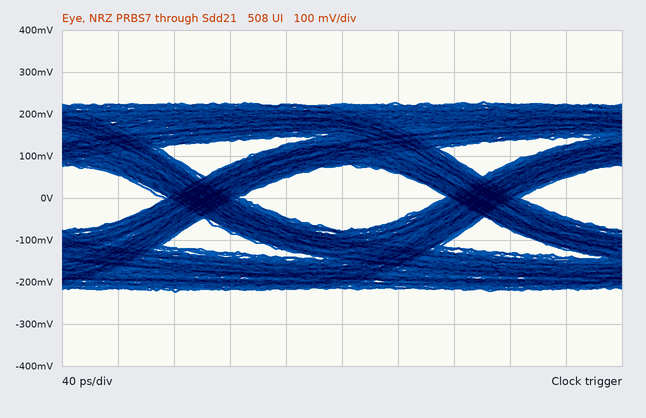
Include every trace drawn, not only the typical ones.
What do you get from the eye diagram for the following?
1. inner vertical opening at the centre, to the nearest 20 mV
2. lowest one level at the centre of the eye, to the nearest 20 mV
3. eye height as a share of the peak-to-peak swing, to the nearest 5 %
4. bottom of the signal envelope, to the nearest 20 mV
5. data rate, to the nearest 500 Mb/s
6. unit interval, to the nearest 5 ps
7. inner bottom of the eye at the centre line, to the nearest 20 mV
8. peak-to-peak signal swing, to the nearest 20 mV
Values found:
160 mV
80 mV
35 %
-220 mV
5.0 Gb/s
200 ps
-80 mV
460 mV
